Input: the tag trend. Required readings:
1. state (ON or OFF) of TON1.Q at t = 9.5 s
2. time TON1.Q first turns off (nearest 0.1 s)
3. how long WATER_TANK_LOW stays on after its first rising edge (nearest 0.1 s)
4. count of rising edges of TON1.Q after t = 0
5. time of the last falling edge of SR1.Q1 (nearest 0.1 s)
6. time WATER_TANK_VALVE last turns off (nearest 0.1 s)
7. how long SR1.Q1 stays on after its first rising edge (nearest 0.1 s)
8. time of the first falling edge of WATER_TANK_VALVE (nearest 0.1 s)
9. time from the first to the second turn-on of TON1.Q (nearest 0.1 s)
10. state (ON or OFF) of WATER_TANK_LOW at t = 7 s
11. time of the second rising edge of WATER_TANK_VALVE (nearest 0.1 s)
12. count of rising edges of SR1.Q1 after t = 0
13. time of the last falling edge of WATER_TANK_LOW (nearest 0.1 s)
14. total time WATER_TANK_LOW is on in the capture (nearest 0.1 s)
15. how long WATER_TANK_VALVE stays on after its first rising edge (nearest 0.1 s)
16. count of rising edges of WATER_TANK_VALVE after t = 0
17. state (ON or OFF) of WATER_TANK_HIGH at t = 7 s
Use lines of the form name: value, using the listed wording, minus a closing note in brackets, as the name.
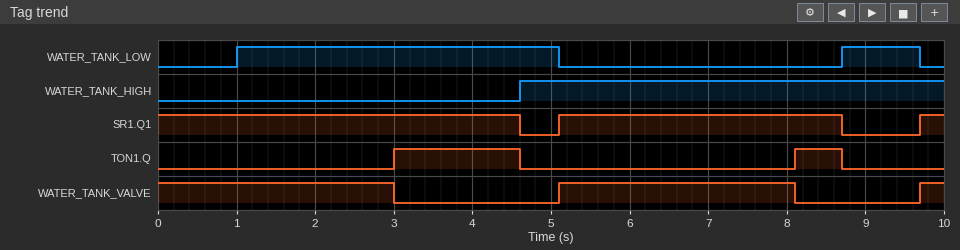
state (ON or OFF) of TON1.Q at t = 9.5 s: OFF
time TON1.Q first turns off: 4.6 s
how long WATER_TANK_LOW stays on after its first rising edge: 4.1 s
count of rising edges of TON1.Q after t = 0: 2
time of the last falling edge of SR1.Q1: 8.7 s
time WATER_TANK_VALVE last turns off: 8.1 s
how long SR1.Q1 stays on after its first rising edge: 3.6 s
time of the first falling edge of WATER_TANK_VALVE: 3.0 s
time from the first to the second turn-on of TON1.Q: 5.1 s
state (ON or OFF) of WATER_TANK_LOW at t = 7 s: OFF
time of the second rising edge of WATER_TANK_VALVE: 9.7 s
count of rising edges of SR1.Q1 after t = 0: 2
time of the last falling edge of WATER_TANK_LOW: 9.7 s
total time WATER_TANK_LOW is on in the capture: 5.1 s
how long WATER_TANK_VALVE stays on after its first rising edge: 3.0 s
count of rising edges of WATER_TANK_VALVE after t = 0: 2
state (ON or OFF) of WATER_TANK_HIGH at t = 7 s: ON
